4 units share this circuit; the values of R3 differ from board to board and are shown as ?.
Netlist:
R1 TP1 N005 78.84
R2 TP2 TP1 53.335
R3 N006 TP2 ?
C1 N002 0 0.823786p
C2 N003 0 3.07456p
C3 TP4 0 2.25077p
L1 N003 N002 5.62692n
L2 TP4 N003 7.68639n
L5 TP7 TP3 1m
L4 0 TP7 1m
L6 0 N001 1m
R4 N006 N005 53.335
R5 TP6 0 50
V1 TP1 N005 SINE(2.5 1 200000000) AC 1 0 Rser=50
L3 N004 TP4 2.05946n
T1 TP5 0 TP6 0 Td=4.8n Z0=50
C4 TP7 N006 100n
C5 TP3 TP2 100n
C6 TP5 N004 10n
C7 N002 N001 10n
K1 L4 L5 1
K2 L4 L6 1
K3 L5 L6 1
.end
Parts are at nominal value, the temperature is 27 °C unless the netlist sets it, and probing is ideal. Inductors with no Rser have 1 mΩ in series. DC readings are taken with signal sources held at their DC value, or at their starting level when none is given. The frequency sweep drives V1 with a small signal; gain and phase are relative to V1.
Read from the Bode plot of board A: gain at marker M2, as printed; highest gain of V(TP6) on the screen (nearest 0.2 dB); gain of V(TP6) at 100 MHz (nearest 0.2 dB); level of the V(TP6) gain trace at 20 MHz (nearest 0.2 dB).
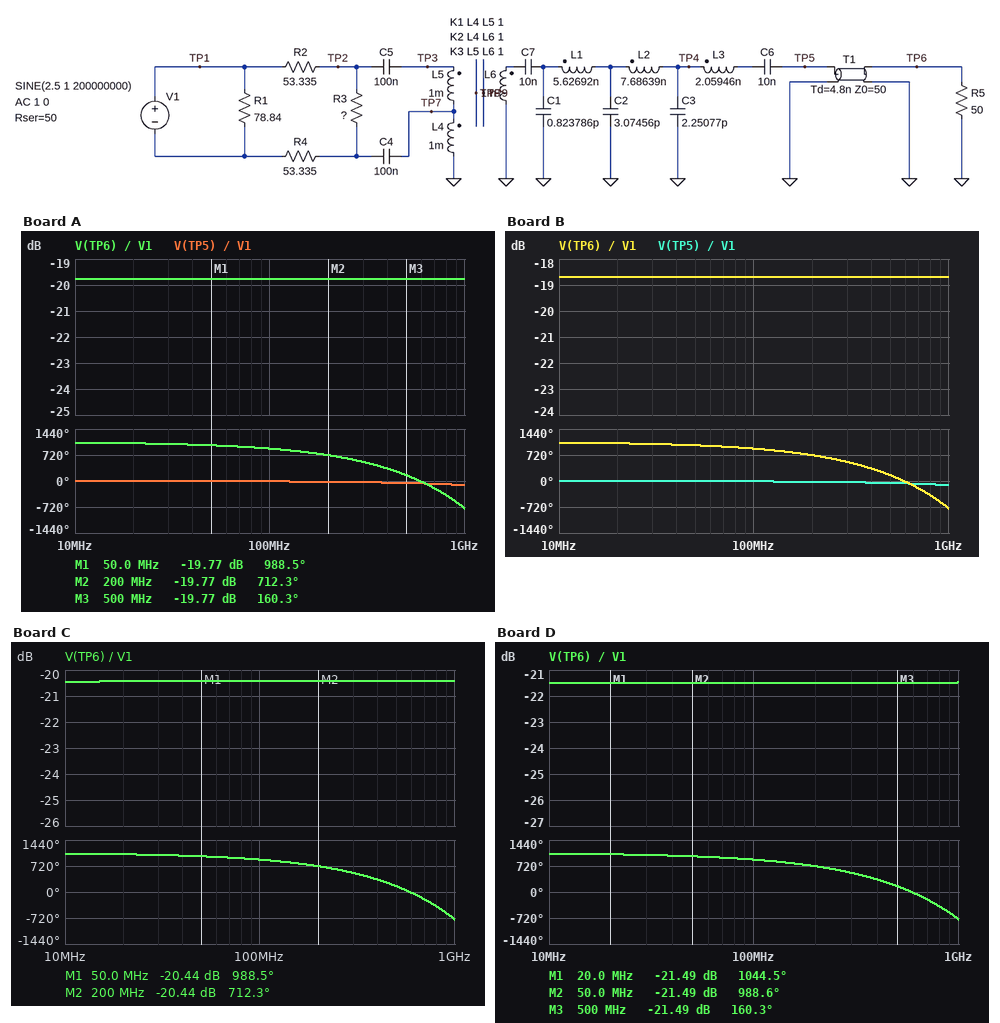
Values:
-19.77 dB
-19.8 dB
-19.8 dB
-19.8 dB
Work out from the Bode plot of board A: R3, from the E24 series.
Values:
62 Ω
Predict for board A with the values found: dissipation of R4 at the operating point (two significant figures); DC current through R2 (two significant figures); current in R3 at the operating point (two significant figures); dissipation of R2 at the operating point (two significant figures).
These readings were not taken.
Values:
3.1 mW
7.7 mA
7.7 mA
3.1 mW
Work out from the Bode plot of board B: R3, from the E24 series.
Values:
91 Ω
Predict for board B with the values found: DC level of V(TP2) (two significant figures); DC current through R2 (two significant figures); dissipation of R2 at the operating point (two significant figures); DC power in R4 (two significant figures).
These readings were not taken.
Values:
310 mV
6.7 mA
2.4 mW
2.4 mW
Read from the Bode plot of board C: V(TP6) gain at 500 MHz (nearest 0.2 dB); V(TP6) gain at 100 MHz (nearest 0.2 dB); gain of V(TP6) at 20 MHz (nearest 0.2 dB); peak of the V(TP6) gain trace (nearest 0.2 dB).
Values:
-20.4 dB
-20.4 dB
-20.4 dB
-20.4 dB
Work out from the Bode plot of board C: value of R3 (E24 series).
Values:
51 Ω
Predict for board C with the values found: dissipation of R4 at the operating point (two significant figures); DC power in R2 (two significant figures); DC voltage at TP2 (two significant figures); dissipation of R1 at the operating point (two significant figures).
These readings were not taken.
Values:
3.5 mW
3.5 mW
210 mV
21 mW
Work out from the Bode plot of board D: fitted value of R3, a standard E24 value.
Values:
39 Ω
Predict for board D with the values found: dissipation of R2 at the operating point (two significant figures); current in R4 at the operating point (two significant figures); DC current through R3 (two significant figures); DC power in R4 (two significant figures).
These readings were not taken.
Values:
4.0 mW
8.7 mA
8.7 mA
4.0 mW
